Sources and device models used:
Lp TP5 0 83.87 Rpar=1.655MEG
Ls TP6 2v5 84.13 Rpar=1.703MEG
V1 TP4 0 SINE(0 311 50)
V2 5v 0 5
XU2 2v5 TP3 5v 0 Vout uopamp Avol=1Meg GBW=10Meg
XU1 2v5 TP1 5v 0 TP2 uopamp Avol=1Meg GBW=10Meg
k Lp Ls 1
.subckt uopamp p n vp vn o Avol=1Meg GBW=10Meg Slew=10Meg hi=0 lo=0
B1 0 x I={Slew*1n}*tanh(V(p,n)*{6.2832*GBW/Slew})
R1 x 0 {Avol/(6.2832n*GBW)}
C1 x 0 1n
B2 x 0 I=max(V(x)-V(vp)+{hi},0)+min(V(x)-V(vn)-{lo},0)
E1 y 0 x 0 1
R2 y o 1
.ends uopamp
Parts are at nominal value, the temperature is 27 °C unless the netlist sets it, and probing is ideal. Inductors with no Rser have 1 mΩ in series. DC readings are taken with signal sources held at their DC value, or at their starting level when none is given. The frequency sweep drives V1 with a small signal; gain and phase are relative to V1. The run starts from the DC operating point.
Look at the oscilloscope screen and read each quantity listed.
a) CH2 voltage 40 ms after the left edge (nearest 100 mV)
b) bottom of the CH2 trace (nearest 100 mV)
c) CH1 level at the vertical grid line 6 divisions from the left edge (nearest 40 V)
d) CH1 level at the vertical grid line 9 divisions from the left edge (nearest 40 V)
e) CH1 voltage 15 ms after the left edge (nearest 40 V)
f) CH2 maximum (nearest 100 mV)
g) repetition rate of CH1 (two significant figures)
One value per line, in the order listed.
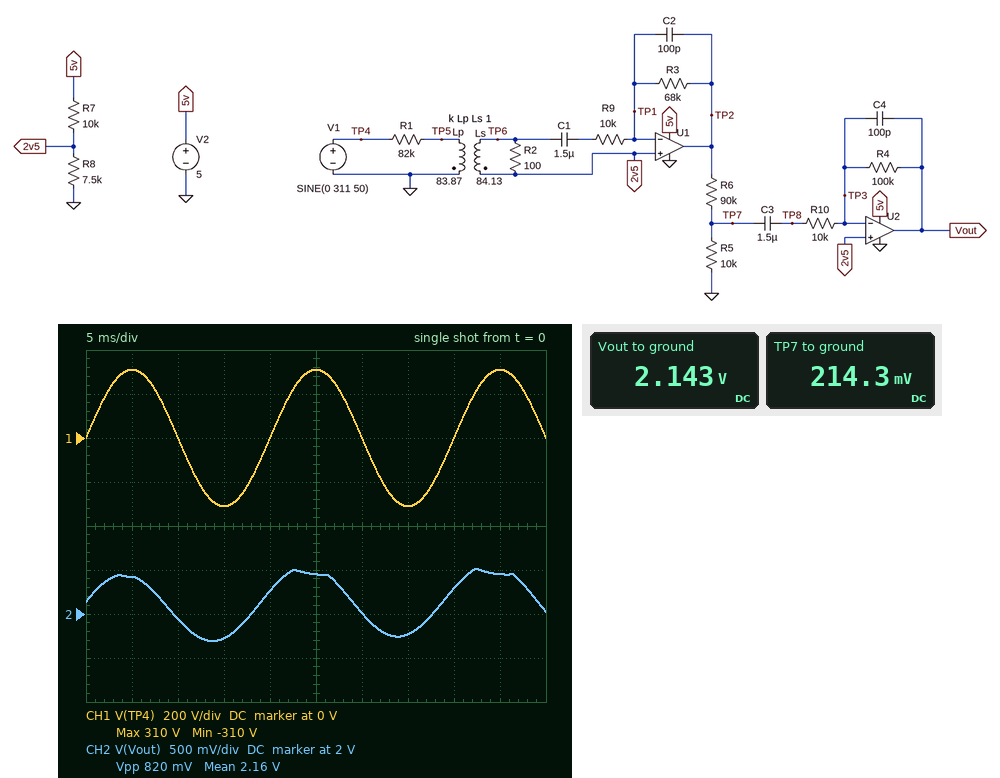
2.3 V
1.7 V
0 V
320 V
-320 V
2.5 V
50 Hz
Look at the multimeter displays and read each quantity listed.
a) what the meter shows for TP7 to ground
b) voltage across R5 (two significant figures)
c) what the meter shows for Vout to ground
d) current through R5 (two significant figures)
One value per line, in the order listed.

214.3 mV
210 mV
2.143 V
21 µA
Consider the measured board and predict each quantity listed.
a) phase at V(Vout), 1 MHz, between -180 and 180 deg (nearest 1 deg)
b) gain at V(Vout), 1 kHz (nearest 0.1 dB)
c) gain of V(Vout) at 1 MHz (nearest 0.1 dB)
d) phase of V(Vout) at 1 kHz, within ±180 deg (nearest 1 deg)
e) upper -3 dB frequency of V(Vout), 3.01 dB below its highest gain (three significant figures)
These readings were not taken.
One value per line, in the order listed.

168 deg
-57.4 dB
-66.0 dB
-12 deg
45.0 kHz
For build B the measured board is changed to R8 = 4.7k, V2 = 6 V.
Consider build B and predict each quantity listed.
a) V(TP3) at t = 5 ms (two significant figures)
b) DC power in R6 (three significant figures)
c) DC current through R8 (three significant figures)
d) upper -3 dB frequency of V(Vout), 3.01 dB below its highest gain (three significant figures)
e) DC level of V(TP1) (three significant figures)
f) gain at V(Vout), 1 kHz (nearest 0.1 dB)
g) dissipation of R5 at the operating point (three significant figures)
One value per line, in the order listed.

1.8 V
33.1 µW
408 µA
24.3 kHz
1.92 V
-53.6 dB
3.68 µW
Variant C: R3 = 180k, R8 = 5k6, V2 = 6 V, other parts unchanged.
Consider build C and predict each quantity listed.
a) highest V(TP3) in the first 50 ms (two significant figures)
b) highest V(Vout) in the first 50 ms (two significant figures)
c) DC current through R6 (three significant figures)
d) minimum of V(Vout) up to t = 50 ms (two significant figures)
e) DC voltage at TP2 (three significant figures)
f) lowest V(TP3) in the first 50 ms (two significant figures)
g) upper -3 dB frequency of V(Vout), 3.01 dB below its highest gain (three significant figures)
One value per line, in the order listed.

2.2 V
3.3 V
21.5 µA
450 mV
2.15 V
2.1 V
7.78 kHz
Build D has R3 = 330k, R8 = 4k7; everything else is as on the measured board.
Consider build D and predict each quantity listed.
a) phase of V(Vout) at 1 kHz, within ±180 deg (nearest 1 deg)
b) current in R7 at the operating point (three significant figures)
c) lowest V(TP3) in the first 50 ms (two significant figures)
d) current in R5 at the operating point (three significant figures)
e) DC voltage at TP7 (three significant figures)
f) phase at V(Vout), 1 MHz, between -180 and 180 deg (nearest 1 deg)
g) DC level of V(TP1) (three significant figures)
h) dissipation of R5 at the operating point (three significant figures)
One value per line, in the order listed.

-16 deg
340 µA
1.6 V
16.0 µA
160 mV
168 deg
1.60 V
2.56 µW
